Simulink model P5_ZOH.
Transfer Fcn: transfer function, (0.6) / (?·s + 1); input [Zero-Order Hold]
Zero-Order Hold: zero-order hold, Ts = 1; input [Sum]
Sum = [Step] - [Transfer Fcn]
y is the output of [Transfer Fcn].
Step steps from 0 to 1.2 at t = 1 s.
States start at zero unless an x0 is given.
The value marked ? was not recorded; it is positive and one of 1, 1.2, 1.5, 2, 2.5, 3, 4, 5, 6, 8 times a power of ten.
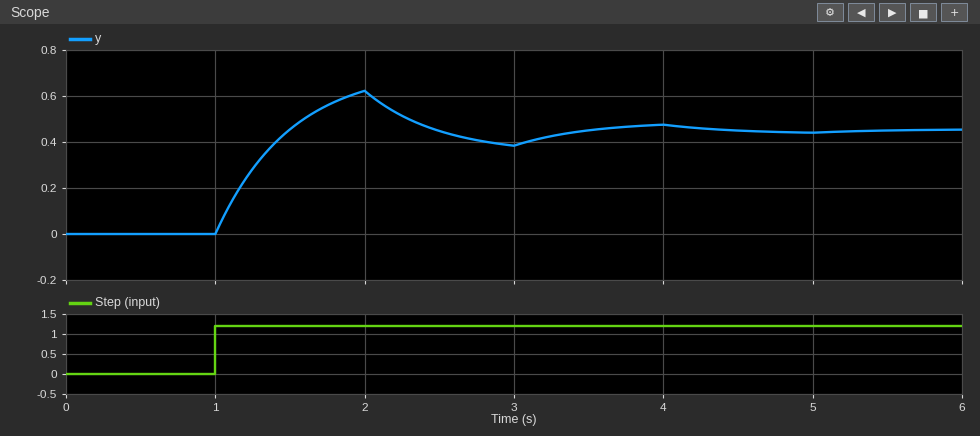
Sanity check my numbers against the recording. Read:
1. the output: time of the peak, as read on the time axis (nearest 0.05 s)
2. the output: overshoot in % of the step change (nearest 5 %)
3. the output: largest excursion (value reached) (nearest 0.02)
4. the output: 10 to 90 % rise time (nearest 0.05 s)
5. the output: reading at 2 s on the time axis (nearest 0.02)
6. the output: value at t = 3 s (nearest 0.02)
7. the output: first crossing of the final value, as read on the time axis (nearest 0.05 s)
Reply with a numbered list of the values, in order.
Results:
1. 2.00 s
2. 40 %
3. 0.62
4. 0.40 s
5. 0.62
6. 0.38
7. 1.50 s
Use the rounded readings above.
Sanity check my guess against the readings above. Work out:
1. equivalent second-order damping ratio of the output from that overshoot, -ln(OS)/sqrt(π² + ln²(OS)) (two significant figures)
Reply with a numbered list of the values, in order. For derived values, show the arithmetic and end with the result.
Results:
1. ln(0.4) = -0.916; 0.916 / sqrt(9.870 + 0.840) = 0.28
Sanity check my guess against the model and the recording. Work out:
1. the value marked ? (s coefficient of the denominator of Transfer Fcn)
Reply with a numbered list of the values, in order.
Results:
1. 0.5
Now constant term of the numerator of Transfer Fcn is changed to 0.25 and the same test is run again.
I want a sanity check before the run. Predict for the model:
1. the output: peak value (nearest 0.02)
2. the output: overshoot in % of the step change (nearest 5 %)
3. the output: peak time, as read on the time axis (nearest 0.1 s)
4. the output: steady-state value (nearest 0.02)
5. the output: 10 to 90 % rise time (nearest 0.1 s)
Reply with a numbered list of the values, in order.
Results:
1. 0.26
2. 10 %
3. 2.0 s
4. 0.24
5. 0.6 s
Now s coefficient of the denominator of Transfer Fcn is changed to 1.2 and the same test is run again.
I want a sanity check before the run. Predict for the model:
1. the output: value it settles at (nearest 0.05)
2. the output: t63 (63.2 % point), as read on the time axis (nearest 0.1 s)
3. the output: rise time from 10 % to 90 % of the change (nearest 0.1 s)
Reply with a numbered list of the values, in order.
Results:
1. 0.45
2. 1.6 s
3. 0.9 s
